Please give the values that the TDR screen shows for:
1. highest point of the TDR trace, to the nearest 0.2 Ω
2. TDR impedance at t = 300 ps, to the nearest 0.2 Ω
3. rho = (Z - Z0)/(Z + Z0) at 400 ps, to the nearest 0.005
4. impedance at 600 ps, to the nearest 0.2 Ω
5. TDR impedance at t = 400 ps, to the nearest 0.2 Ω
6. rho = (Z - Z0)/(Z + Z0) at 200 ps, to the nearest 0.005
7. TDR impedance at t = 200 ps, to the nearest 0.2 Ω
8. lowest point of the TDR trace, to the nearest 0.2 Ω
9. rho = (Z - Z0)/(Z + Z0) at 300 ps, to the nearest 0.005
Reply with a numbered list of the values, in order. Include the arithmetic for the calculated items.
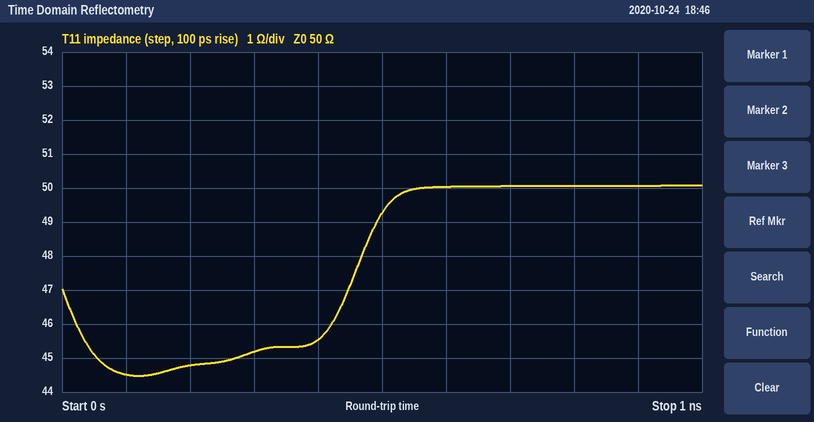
1. 50.0 Ω
2. 45.2 Ω
3. (45.6 − 50)/(45.6 + 50) ≈ -0.0460, so -0.045 to the nearest 0.005
4. 50.0 Ω
5. 45.6 Ω
6. (44.8 − 50)/(44.8 + 50) ≈ -0.055
7. 44.8 Ω
8. 44.4 Ω
9. (45.2 − 50)/(45.2 + 50) ≈ -0.050
